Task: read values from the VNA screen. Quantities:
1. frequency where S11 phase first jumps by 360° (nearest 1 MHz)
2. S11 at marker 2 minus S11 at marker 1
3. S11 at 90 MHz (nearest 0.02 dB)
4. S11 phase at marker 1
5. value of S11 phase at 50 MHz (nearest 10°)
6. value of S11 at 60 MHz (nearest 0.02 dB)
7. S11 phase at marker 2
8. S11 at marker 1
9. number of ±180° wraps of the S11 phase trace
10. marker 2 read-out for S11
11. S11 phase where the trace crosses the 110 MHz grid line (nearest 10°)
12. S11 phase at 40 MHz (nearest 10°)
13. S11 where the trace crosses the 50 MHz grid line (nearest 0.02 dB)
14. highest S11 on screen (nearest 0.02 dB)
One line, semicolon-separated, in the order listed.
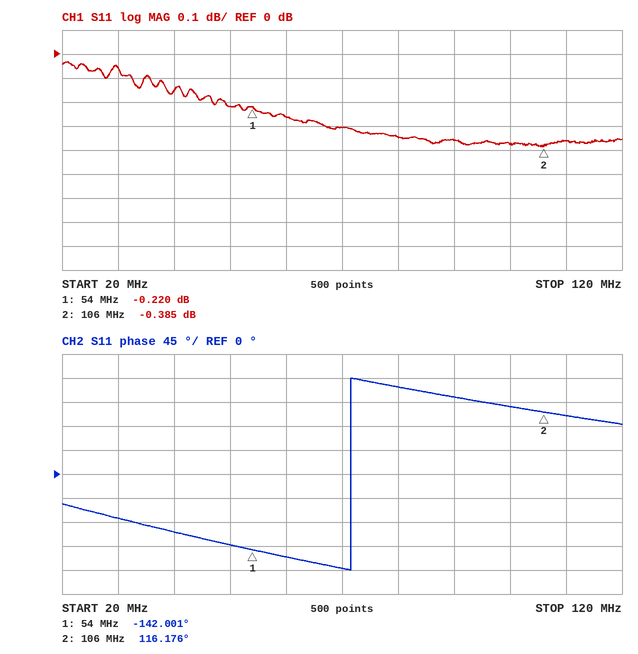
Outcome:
72 MHz; -0.165 dB; -0.36 dB; -142.001°; -130°; -0.26 dB; 116.176°; -0.220 dB; 1; -0.385 dB; 110°; -110°; -0.22 dB; -0.04 dB
